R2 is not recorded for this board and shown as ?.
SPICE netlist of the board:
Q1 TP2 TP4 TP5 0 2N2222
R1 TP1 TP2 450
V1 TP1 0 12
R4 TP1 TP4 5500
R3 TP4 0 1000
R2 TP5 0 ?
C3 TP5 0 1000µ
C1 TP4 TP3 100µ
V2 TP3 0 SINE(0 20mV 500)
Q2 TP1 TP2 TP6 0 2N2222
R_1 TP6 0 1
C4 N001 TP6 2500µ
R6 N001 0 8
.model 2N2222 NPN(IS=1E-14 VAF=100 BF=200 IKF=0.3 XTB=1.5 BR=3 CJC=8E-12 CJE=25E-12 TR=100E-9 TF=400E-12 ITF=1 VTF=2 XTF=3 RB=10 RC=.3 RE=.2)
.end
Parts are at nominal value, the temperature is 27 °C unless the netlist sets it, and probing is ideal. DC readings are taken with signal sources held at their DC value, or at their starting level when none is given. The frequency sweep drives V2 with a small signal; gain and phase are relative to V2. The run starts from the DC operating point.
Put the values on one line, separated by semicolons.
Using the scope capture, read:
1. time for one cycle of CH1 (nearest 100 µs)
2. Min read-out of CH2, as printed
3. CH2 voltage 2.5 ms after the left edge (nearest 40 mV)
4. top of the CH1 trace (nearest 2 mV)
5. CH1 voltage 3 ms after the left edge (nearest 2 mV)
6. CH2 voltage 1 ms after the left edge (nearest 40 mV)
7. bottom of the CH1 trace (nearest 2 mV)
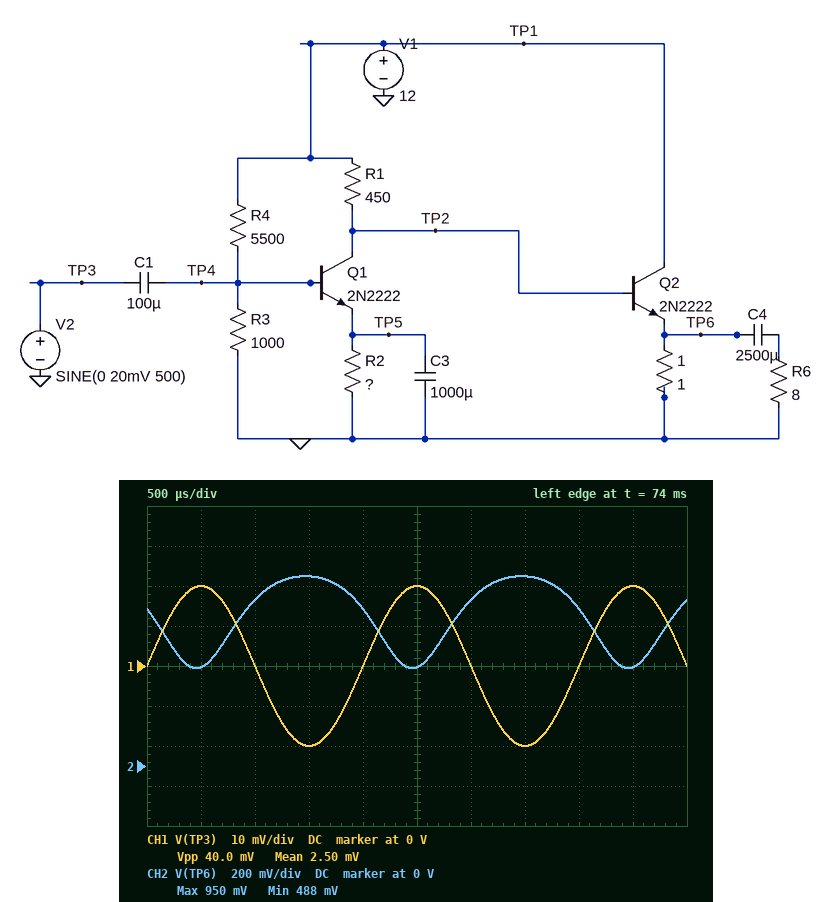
2.0 ms; 488 mV; 480 mV; 20 mV; 0 V; 840 mV; -20 mV
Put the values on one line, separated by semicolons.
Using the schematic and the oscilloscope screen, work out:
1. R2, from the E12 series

100 Ω
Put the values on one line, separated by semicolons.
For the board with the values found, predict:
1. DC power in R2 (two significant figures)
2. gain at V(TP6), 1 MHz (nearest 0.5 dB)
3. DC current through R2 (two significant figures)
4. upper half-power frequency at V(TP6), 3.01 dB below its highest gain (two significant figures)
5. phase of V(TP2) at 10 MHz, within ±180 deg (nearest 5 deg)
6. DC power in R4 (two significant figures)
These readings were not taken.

12 mW; 21.0 dB; 11 mA; 9.1 MHz; 135 deg; 19 mW
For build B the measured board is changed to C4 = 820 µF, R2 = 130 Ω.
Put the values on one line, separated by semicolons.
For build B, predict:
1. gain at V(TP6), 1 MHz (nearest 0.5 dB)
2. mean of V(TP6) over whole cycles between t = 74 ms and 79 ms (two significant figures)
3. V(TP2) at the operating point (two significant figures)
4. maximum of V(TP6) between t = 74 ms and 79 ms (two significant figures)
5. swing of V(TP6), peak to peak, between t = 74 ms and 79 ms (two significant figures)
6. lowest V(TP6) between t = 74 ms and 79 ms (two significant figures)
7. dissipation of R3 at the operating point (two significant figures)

18.5 dB; 850 mV; 2.0 V; 990 mV; 340 mV; 650 mV; 3.3 mW
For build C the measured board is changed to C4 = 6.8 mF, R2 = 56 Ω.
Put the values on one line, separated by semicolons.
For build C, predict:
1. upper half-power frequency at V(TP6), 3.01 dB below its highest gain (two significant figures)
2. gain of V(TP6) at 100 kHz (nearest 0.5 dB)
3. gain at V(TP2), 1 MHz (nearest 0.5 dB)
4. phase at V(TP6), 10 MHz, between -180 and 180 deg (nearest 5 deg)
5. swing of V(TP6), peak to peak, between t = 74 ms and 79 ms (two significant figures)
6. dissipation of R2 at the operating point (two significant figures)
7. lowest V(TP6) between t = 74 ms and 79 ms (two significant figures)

6.2 MHz; 28.0 dB; 31.5 dB; 115 deg; 610 mV; 19 mW; 210 mV
